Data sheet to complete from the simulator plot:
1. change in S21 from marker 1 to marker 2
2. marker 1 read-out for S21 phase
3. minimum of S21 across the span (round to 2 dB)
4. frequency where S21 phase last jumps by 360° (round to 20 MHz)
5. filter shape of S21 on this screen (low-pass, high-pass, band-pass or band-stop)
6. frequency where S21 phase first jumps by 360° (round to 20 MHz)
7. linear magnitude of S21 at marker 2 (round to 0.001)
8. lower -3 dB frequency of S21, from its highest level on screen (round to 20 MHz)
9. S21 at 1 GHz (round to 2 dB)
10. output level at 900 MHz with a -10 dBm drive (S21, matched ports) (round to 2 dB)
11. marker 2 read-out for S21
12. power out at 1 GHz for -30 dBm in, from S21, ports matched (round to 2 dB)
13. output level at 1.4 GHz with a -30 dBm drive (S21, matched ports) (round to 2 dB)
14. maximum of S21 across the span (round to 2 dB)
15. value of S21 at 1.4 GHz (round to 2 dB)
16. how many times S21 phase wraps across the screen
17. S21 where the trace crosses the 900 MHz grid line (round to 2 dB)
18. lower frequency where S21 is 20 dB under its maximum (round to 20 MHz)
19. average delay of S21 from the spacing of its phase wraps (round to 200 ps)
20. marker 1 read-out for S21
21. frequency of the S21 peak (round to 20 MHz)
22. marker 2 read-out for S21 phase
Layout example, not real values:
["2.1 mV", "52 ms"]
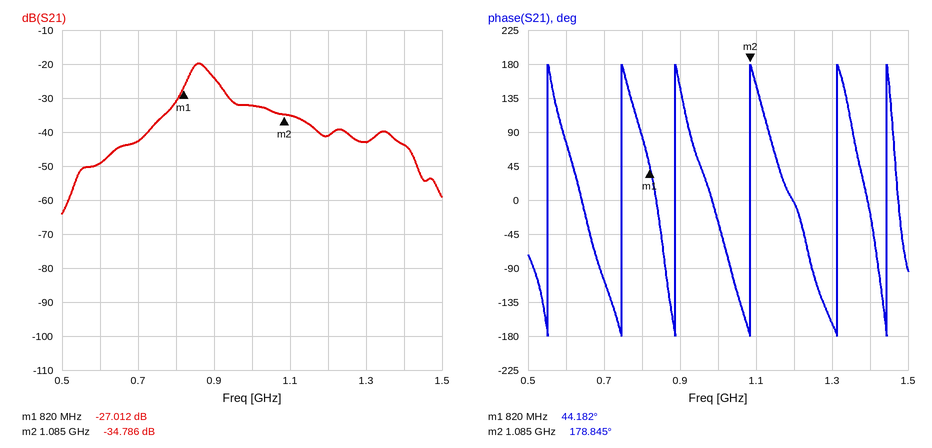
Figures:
["-7.774 dB", "44.182°", "-64 dB", "1.44 GHz", "band-pass", "560 MHz", "0.018", "840 MHz", "-32 dB", "-34 dBm", "-34.786 dB", "-62 dBm", "-74 dBm", "-20 dB", "-44 dB", "6", "-24 dB", "720 MHz", "5.6 ns", "-27.012 dB", "860 MHz", "178.845°"]
